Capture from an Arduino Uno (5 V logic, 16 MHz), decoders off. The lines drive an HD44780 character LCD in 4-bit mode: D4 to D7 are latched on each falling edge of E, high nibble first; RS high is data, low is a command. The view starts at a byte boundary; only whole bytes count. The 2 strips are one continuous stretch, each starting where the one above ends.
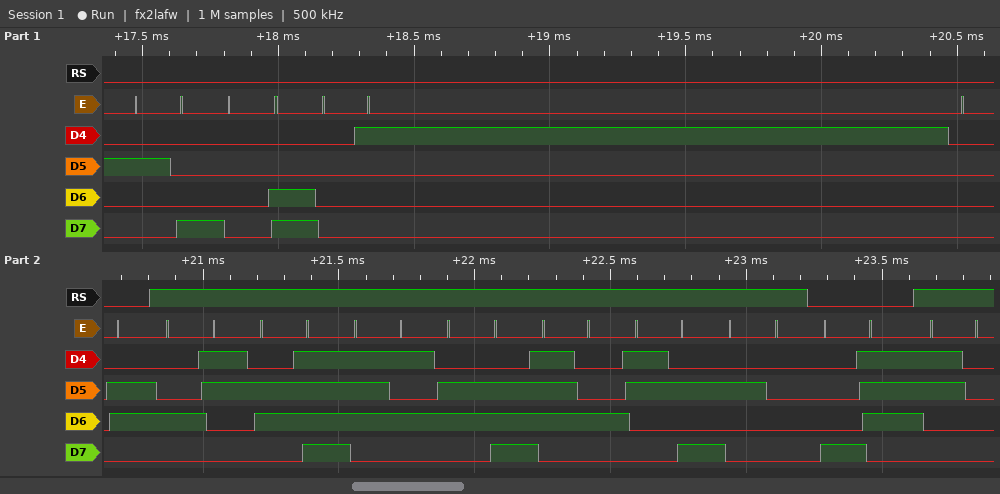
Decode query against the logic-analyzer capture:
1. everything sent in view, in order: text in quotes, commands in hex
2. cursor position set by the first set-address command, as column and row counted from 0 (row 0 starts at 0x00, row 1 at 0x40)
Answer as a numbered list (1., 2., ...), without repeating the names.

1. 0x28 0x0C 0x01 0x06 "Count: " 0x87 "0"
2. column 7, row 0
